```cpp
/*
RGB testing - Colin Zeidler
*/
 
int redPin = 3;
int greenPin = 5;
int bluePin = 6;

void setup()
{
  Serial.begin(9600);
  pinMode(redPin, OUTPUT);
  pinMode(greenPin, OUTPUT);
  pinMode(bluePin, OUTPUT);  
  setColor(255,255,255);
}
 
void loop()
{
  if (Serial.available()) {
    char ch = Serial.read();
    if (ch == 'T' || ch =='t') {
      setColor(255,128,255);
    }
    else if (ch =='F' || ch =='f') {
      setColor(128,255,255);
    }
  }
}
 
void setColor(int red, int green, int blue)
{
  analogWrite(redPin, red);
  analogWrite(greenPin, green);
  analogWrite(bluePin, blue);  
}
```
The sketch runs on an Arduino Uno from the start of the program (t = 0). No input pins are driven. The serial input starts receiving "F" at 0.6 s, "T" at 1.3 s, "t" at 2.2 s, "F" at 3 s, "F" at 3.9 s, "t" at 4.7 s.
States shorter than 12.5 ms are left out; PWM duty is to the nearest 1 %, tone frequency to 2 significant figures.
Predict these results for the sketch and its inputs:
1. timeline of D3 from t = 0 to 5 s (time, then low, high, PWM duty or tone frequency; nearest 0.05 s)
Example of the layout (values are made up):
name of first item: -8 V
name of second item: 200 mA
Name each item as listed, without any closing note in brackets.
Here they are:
timeline of D3 from t = 0 to 5 s: 0 s high; 0.6 s PWM 50 %; 1.3 s high; 3 s PWM 50 %; 4.7 s high
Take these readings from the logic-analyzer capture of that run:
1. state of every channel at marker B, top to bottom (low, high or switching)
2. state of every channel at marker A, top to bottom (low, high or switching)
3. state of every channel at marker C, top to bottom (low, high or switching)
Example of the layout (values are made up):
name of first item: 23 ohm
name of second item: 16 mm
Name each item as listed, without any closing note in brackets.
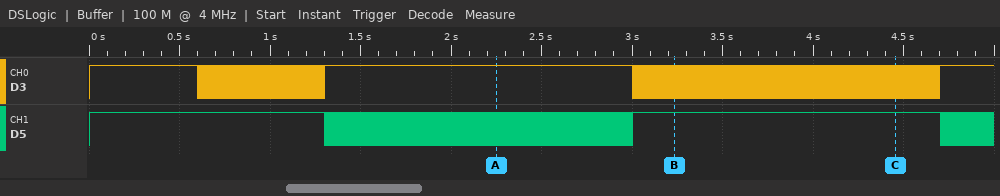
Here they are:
state of every channel at marker B, top to bottom: D3 switching, D5 high
state of every channel at marker A, top to bottom: D3 high, D5 switching
state of every channel at marker C, top to bottom: D3 switching, D5 high
